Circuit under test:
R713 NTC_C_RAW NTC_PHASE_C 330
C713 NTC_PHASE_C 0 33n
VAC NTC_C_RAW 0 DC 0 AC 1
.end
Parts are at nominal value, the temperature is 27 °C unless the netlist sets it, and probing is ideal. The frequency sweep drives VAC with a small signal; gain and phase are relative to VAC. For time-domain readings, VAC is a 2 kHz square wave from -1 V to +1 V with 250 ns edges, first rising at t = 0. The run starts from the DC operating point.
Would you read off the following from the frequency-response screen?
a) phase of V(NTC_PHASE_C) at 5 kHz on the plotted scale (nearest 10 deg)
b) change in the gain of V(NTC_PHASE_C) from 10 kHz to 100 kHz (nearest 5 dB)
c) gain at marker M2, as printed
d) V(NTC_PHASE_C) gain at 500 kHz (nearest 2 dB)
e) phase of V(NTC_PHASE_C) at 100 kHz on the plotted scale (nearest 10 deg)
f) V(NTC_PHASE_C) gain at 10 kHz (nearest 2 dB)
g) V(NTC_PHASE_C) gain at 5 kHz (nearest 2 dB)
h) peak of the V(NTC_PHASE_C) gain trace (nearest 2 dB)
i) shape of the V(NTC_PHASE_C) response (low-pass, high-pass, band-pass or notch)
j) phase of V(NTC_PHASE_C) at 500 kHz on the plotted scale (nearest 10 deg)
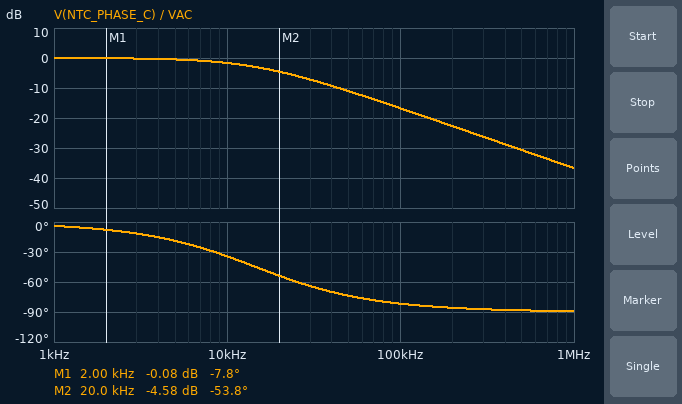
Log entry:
-20 deg
-15 dB
-4.58 dB
-30 dB
-80 deg
-2 dB
0 dB
0 dB
low-pass
-90 deg
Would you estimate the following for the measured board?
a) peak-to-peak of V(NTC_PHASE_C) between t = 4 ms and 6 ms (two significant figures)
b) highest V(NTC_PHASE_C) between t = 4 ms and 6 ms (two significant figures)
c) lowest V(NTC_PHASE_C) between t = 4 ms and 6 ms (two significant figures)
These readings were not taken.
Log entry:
2.0 V
1.0 V
-1.0 V
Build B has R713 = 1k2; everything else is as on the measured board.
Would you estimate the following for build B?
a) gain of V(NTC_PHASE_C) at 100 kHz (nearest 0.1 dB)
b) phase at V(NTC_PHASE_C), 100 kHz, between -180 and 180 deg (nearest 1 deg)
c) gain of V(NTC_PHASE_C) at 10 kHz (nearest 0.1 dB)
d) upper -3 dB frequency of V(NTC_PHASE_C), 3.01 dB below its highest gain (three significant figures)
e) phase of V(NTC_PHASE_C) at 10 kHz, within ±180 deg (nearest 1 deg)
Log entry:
-27.9 dB
-88 deg
-8.6 dB
4.02 kHz
-68 deg
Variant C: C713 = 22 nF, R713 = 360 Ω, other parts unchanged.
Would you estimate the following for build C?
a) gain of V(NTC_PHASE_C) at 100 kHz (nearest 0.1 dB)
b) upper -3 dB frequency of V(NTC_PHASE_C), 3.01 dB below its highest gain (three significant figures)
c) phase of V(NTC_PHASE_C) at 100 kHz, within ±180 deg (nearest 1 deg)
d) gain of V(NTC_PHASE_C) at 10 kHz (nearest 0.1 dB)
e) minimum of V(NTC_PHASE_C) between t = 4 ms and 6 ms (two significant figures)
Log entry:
-14.1 dB
20.1 kHz
-79 deg
-1.0 dB
-1.0 V
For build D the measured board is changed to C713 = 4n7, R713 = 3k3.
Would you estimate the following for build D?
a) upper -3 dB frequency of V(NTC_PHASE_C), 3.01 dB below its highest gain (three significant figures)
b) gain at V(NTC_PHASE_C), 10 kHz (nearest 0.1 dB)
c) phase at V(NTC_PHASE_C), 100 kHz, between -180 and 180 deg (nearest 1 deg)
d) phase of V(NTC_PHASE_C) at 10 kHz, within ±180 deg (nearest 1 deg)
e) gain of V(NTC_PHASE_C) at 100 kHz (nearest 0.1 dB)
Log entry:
10.3 kHz
-2.9 dB
-84 deg
-44 deg
-19.8 dB
